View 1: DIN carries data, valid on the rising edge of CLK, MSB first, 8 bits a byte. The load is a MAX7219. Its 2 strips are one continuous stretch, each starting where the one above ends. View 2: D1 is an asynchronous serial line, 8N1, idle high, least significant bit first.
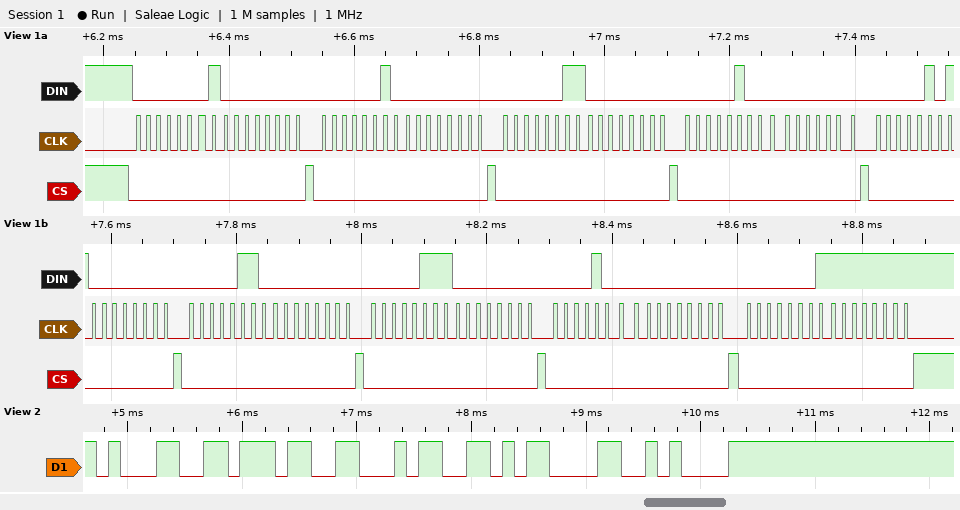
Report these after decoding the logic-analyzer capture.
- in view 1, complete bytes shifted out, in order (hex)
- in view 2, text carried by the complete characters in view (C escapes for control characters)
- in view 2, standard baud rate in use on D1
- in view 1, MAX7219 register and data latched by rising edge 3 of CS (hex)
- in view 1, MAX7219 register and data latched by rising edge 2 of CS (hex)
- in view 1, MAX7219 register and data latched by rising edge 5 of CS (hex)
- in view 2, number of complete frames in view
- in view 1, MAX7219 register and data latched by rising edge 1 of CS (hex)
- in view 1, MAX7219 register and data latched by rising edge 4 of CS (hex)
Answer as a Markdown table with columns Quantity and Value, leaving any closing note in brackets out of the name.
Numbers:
| Quantity | Value |
|---|---|
| in view 1, complete bytes shifted out, in order | 01 00 02 00 03 00 04 00 05 00 06 00 07 00 08 00 01 FF |
| in view 2, text carried by the complete characters in view | "174\r\n" |
| in view 2, standard baud rate in use on D1 | 9600 baud |
| in view 1, MAX7219 register and data latched by rising edge 3 of CS | register 0x3, data 0x00 |
| in view 1, MAX7219 register and data latched by rising edge 2 of CS | register 0x2, data 0x00 |
| in view 1, MAX7219 register and data latched by rising edge 5 of CS | register 0x5, data 0x00 |
| in view 2, number of complete frames in view | 5 |
| in view 1, MAX7219 register and data latched by rising edge 1 of CS | register 0x1, data 0x00 |
| in view 1, MAX7219 register and data latched by rising edge 4 of CS | register 0x4, data 0x00 |
